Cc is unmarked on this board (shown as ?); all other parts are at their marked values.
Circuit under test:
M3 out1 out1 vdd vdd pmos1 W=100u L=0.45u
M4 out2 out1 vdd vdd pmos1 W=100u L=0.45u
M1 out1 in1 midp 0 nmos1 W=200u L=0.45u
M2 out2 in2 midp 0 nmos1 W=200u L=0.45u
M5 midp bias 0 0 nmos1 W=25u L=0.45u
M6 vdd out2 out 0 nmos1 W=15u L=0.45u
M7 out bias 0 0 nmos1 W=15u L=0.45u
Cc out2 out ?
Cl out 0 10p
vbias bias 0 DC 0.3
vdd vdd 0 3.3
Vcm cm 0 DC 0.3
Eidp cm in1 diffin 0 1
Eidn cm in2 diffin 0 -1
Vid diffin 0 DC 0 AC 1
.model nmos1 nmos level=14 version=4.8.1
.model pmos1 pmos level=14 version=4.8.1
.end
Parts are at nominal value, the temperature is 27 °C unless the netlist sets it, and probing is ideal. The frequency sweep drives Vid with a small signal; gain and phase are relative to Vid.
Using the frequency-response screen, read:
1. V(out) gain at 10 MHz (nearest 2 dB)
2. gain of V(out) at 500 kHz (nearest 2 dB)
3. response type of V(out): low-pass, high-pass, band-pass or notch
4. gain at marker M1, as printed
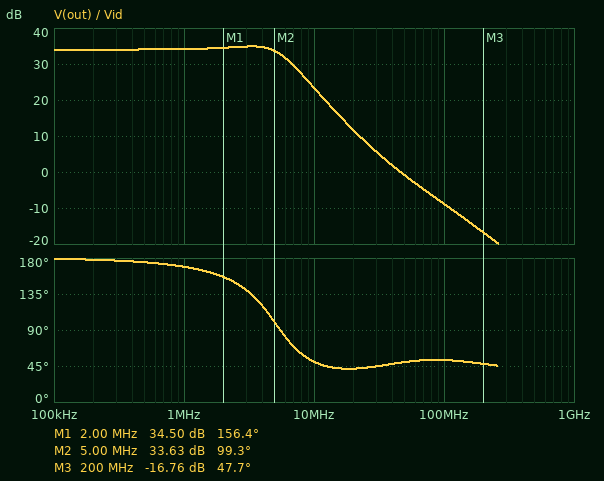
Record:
24 dB
34 dB
low-pass
34.50 dB
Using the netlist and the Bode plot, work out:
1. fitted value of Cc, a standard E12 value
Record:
8.2 pF
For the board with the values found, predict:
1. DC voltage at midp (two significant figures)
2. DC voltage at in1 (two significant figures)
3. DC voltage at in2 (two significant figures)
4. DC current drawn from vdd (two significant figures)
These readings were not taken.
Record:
130 mV
300 mV
300 mV
190 µA
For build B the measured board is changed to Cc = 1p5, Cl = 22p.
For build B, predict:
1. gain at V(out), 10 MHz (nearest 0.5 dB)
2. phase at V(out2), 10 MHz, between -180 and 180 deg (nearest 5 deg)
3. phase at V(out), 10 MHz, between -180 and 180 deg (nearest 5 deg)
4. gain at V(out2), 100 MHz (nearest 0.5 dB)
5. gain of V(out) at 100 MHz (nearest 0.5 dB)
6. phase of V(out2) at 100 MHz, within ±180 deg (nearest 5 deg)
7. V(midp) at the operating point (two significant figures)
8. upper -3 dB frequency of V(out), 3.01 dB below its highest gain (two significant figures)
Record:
28.0 dB
95 deg
60 deg
5.5 dB
-12.0 dB
65 deg
130 mV
7.8 MHz
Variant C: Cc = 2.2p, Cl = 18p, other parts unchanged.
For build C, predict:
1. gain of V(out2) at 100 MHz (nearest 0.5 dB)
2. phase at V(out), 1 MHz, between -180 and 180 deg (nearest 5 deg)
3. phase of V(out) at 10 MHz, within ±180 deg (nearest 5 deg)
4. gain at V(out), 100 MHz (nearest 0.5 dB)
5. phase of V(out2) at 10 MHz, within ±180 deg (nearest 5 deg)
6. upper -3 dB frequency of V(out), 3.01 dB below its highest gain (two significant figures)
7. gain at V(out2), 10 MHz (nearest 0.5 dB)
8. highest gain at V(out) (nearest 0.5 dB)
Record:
3.5 dB
170 deg
55 deg
-11.5 dB
85 deg
7.7 MHz
30.0 dB
34.5 dB
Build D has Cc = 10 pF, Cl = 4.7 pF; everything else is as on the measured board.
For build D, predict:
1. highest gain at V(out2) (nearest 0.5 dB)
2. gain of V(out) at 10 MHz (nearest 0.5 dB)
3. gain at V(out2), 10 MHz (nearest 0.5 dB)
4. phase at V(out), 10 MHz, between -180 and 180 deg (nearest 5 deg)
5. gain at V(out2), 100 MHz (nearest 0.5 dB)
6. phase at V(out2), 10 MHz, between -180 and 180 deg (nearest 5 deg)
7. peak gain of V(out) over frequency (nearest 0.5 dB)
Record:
34.5 dB
26.5 dB
27.5 dB
75 deg
0.5 dB
80 deg
34.0 dB
